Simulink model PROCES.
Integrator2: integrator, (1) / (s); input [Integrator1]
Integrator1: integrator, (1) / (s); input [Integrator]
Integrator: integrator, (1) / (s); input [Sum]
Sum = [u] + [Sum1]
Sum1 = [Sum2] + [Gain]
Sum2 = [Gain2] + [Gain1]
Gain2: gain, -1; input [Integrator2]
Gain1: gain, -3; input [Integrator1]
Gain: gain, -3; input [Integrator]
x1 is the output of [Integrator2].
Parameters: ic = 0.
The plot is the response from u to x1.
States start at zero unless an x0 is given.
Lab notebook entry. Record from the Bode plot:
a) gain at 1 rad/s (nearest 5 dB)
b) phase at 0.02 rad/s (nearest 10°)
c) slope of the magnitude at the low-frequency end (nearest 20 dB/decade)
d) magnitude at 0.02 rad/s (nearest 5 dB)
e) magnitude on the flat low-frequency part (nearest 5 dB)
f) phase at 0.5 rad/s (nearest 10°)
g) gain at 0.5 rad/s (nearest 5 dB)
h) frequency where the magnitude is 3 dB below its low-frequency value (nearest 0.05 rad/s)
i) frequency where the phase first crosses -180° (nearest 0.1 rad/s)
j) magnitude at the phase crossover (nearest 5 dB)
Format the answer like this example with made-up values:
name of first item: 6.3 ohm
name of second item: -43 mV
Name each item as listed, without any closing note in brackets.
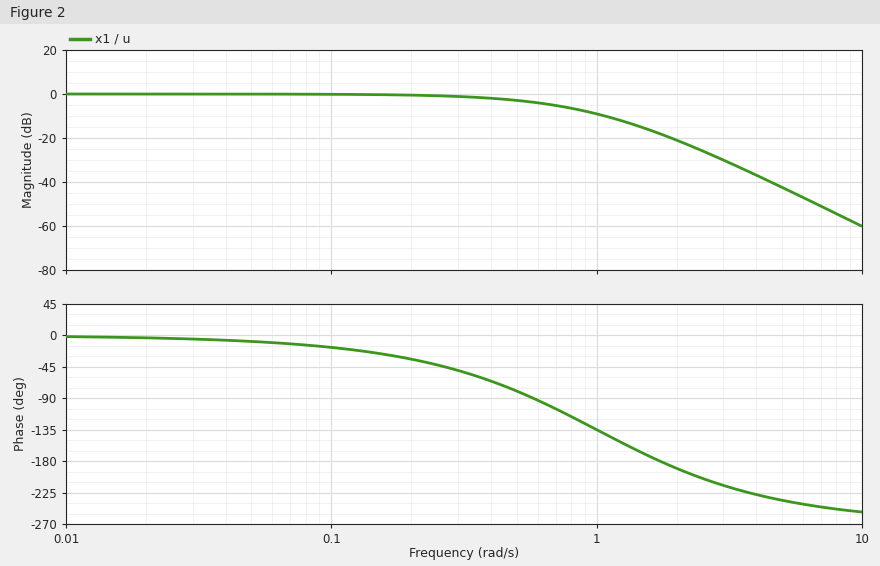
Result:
gain at 1 rad/s: -10 dB
phase at 0.02 rad/s: 0°
slope of the magnitude at the low-frequency end: 0 dB/decade
magnitude at 0.02 rad/s: 0 dB
magnitude on the flat low-frequency part: 0 dB
phase at 0.5 rad/s: -80°
gain at 0.5 rad/s: -5 dB
frequency where the magnitude is 3 dB below its low-frequency value: 0.50 rad/s
frequency where the phase first crosses -180°: 1.7 rad/s
magnitude at the phase crossover: -20 dB
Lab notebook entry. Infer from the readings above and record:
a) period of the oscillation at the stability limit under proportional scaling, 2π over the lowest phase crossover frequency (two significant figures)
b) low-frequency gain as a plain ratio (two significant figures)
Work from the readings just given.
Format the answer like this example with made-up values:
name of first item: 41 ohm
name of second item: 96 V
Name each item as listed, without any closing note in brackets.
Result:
period of the oscillation at the stability limit under proportional scaling, 2π over the lowest phase crossover frequency: 3.7 s
low-frequency gain as a plain ratio: 1.0
